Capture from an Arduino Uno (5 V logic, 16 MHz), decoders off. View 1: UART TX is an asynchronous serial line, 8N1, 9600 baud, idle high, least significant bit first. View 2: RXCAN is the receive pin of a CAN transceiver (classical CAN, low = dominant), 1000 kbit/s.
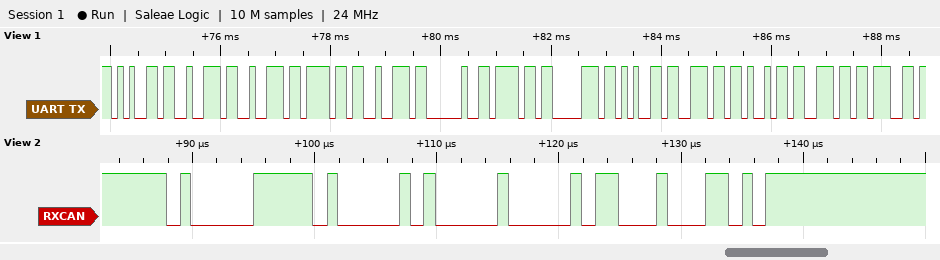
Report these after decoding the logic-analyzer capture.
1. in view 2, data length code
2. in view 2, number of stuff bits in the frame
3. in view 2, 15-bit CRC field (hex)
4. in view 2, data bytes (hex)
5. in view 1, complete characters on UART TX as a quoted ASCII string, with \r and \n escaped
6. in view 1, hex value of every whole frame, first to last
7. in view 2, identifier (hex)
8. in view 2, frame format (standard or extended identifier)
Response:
1
5
0x0C46
00
"error opening"
65 72 72 6F 72 20 6F 70 65 6E 69 6E 67
0x41F
standard
